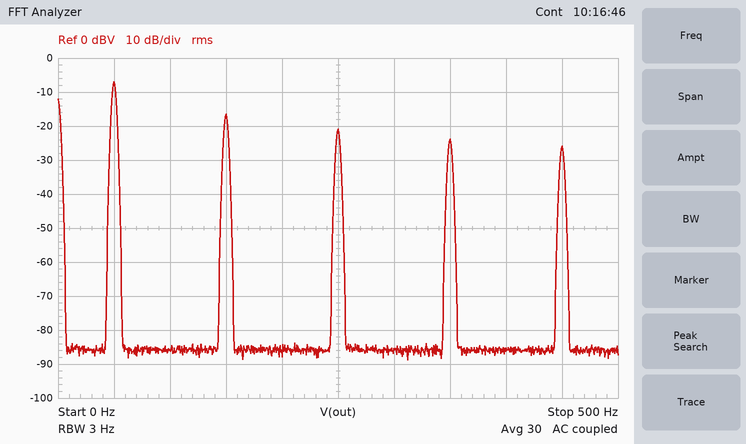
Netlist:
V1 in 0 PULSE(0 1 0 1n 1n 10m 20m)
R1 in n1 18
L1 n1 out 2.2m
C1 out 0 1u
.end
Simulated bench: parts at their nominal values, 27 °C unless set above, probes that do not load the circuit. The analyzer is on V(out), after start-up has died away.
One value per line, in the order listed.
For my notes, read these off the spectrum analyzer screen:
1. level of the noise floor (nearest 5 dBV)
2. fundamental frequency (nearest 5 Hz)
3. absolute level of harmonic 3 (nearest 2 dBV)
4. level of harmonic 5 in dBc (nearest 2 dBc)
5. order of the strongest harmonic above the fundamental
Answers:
-85 dBV
50 Hz
-16 dBV
-14 dBc
3
